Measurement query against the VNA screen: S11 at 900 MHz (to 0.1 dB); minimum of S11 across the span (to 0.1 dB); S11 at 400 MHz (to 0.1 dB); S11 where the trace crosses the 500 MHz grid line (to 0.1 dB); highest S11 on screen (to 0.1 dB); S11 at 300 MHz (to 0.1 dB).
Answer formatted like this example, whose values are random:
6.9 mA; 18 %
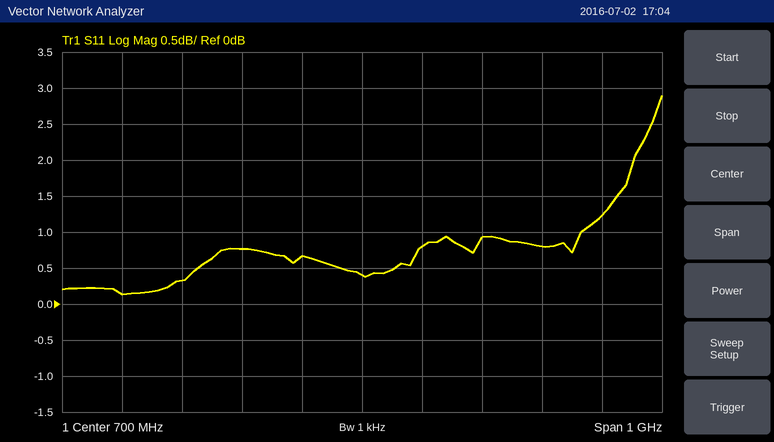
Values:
0.9 dB; 0.1 dB; 0.3 dB; 0.8 dB; 2.9 dB; 0.1 dB
